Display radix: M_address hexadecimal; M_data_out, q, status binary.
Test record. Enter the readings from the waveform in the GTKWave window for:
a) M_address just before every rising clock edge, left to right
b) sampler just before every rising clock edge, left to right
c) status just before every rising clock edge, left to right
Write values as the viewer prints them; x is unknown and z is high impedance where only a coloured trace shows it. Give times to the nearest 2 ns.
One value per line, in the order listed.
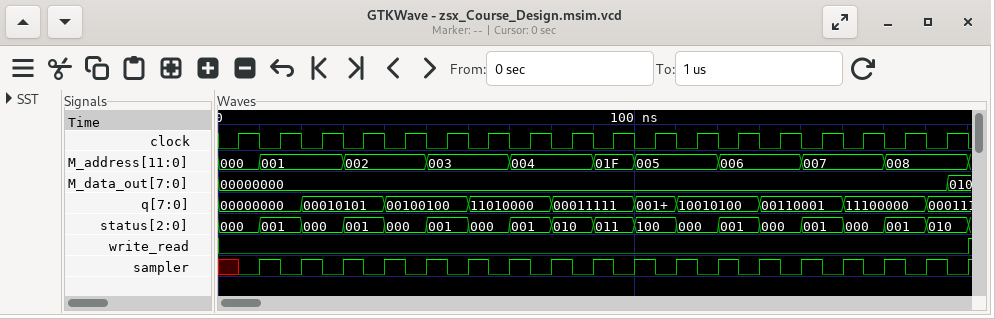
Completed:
000, 001, 001, 002, 002, 003, 003, 004, 004, 01F, 005, 005, 006, 006, 007, 007, 008, 008
x 1 1 1 1 1 1 1 1 1 1 1 1 1 1 1 1 1
000, 001, 000, 001, 000, 001, 000, 001, 010, 011, 100, 000, 001, 000, 001, 000, 001, 010
